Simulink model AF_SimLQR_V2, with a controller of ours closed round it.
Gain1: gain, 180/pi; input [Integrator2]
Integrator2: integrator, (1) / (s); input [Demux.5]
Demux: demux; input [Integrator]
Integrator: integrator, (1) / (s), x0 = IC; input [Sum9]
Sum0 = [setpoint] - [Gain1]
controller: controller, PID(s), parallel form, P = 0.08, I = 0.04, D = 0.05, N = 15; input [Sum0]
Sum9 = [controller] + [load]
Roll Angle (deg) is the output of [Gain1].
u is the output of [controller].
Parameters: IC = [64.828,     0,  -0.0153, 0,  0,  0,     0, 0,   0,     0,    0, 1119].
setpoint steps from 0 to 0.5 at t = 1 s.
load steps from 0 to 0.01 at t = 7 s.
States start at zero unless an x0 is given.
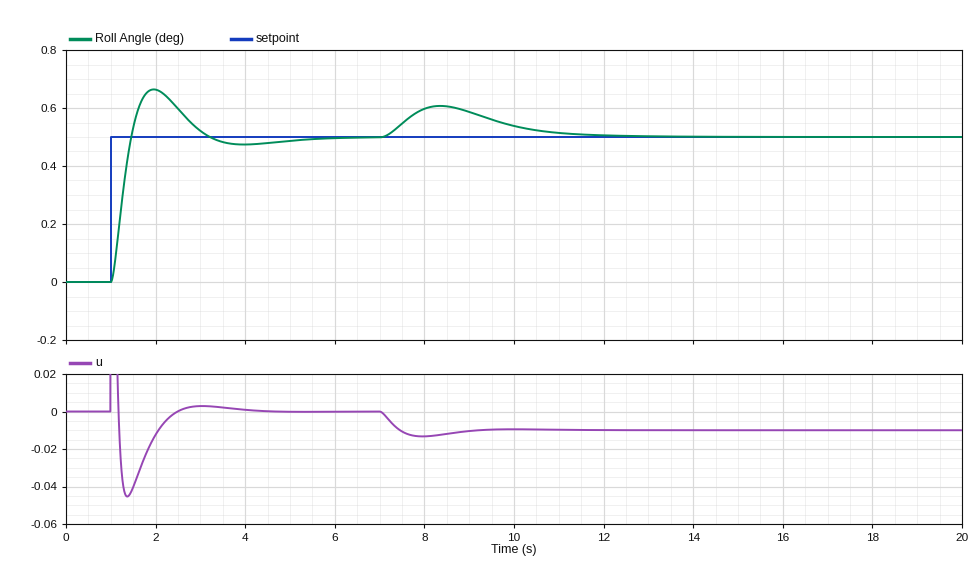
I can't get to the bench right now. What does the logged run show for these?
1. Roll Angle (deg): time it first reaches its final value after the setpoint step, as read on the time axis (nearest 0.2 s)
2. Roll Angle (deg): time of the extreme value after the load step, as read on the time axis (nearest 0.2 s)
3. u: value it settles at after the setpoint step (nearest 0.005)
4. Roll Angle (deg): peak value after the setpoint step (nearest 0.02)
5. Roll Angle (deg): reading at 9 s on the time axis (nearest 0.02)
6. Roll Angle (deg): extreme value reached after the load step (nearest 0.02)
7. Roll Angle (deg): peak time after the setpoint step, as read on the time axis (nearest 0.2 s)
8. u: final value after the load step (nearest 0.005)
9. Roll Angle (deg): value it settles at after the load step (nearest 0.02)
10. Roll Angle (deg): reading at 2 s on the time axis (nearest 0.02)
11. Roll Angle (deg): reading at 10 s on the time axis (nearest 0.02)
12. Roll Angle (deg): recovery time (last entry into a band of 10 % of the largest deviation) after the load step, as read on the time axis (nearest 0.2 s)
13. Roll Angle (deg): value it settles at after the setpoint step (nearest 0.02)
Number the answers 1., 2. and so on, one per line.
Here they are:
1. 1.4 s
2. 8.4 s
3. 0.000
4. 0.66
5. 0.58
6. 0.60
7. 2.0 s
8. -0.010
9. 0.50
10. 0.66
11. 0.54
12. 11.2 s
13. 0.50
